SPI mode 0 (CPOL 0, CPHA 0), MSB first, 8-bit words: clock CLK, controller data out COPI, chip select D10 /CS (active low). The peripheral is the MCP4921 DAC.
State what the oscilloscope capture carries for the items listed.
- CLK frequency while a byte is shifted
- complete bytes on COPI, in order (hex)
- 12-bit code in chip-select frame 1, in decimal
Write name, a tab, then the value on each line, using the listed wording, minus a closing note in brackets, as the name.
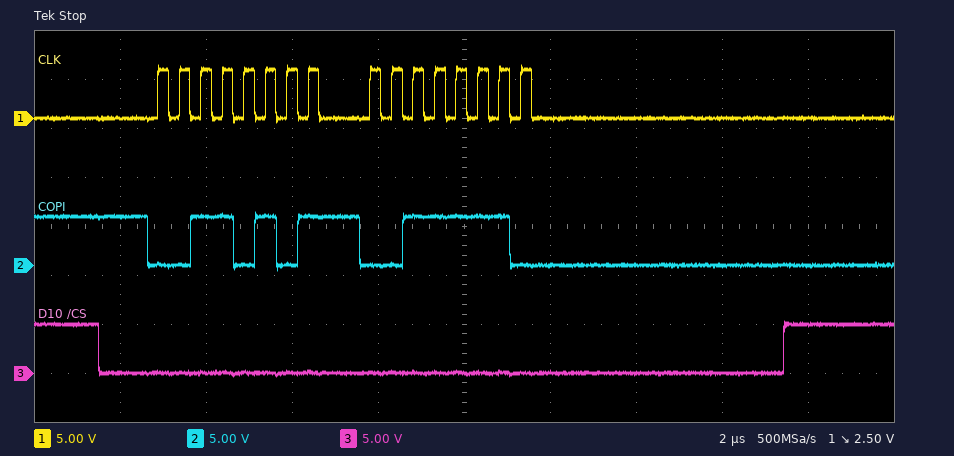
CLK frequency while a byte is shifted	2 MHz
complete bytes on COPI, in order	35 3E
12-bit code in chip-select frame 1, in decimal	1342
